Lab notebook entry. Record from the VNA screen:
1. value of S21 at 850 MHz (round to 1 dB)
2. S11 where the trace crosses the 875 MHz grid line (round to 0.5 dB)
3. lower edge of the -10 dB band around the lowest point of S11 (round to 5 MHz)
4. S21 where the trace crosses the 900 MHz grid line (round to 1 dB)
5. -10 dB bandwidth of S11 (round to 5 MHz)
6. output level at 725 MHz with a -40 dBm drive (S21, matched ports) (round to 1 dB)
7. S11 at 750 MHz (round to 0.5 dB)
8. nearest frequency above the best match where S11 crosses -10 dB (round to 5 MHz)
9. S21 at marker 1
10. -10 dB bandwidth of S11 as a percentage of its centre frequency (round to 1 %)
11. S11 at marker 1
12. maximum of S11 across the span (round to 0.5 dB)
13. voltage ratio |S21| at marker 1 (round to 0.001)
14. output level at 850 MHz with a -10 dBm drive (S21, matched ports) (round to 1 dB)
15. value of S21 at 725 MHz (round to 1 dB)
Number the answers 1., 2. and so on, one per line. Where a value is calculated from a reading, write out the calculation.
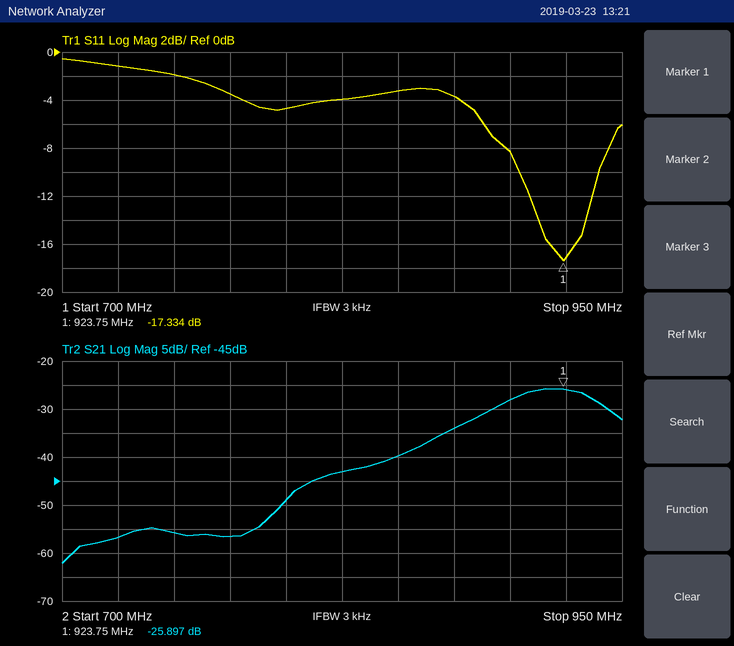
1. -40 dB
2. -3.5 dB
3. 905 MHz
4. -28 dB
5. 940 MHz − 905 MHz = 35 MHz
6. -40 dBm + (-57 dB) = -97 dBm
7. -2.0 dB
8. 940 MHz
9. -25.897 dB
10. 35 MHz / 922.5 MHz ≈ 4 %
11. -17.334 dB
12. -0.5 dB
13. 10^(-25.897/20) ≈ 0.051
14. -10 dBm + (-40 dB) = -50 dBm
15. -57 dB
